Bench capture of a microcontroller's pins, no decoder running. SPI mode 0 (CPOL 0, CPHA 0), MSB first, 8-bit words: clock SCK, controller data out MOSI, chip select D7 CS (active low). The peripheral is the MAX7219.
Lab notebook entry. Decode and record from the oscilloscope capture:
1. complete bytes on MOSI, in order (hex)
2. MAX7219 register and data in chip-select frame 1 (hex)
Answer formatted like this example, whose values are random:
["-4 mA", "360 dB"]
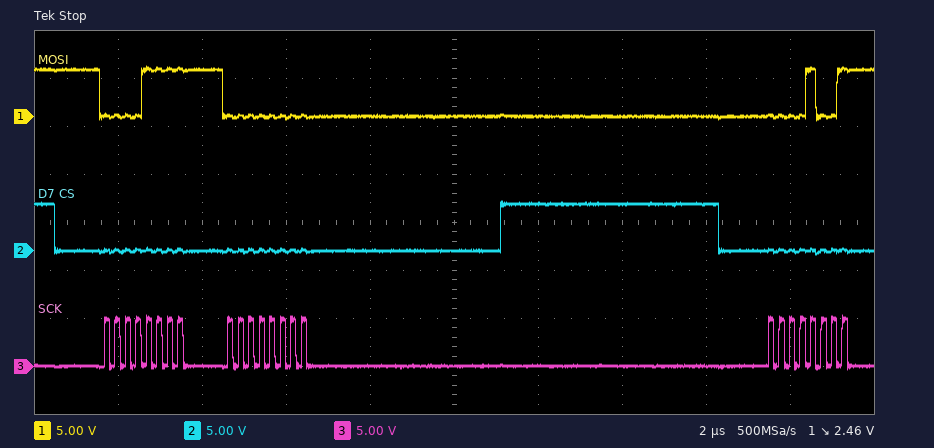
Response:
["0x0F 0x00 0x09", "register 0xF, data 0x00"]
